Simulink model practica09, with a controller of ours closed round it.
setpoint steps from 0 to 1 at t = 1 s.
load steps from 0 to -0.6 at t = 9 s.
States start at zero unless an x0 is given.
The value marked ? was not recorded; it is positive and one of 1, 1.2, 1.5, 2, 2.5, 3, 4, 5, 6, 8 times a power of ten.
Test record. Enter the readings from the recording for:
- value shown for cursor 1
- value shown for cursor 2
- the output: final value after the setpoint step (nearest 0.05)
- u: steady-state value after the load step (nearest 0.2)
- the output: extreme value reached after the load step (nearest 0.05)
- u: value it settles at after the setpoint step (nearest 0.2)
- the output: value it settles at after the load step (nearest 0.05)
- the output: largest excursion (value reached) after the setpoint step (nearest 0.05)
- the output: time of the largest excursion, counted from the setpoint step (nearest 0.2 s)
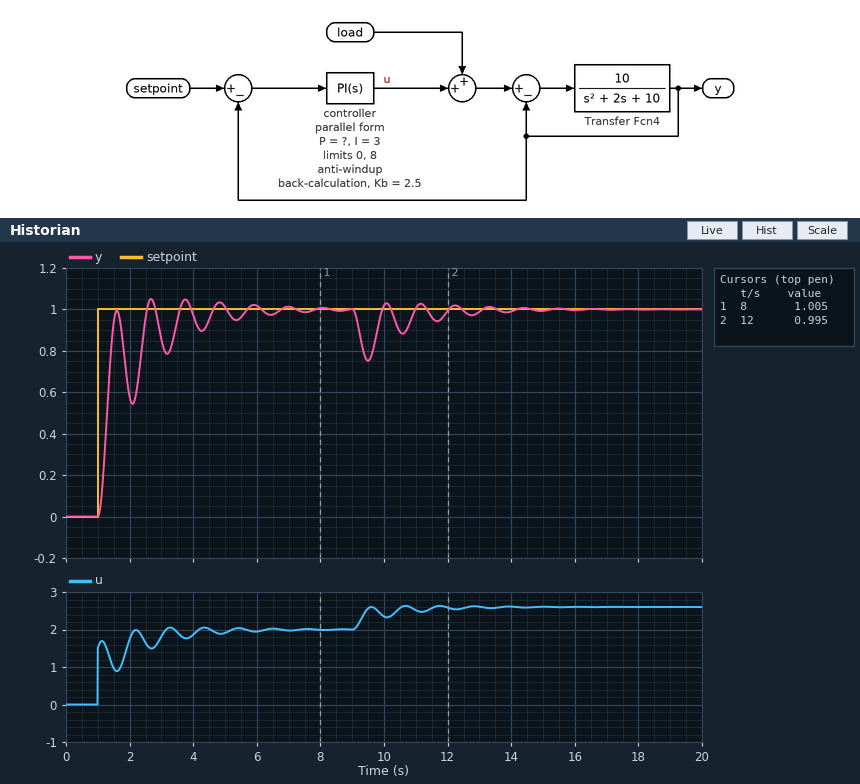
1.005
0.995
1.00
2.6
0.75
2.0
1.00
1.05
1.6 s
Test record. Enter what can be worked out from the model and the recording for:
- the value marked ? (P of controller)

1.5
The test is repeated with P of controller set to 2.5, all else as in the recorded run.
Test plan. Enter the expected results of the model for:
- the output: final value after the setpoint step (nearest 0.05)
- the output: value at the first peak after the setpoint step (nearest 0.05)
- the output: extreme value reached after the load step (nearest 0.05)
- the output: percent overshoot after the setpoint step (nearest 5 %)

1.00
1.10
0.80
10 %
